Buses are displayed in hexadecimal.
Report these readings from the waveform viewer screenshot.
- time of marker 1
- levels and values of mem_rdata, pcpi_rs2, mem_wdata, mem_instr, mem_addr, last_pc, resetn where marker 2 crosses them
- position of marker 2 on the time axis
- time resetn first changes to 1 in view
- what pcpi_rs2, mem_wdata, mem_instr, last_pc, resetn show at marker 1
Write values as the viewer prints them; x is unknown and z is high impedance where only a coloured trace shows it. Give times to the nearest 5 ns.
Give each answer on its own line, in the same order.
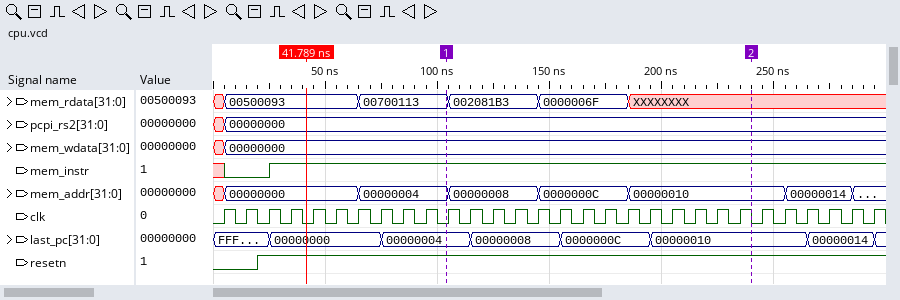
105 ns
mem_rdata=XXXXXXXX, pcpi_rs2=00000000, mem_wdata=00000000, mem_instr=1, mem_addr=00000010, last_pc=00000010, resetn=1
240 ns
20 ns
pcpi_rs2=00000000, mem_wdata=00000000, mem_instr=1, last_pc=00000004, resetn=1
